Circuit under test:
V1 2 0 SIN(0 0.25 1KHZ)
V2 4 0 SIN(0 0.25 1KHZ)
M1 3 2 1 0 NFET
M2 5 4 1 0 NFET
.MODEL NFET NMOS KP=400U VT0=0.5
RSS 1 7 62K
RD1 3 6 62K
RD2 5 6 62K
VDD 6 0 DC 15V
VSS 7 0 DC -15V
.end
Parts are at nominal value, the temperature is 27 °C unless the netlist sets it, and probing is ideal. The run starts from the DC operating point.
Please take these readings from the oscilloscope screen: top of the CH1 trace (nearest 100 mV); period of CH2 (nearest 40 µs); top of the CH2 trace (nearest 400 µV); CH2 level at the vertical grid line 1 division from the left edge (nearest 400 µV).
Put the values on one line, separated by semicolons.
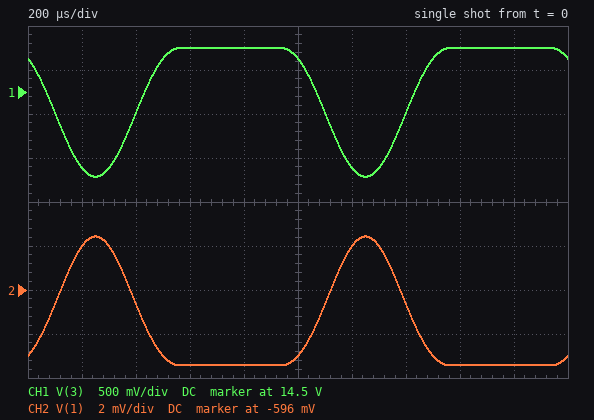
15.0 V; 1.00 ms; -593.6 mV; -594.0 mV
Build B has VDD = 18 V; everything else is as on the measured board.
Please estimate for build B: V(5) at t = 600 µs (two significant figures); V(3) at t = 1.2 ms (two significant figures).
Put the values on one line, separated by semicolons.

18 V; 17 V
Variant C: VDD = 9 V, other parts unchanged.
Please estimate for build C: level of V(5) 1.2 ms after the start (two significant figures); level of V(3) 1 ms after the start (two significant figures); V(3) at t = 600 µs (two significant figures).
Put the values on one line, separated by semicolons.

7.6 V; 8.9 V; 9.0 V
